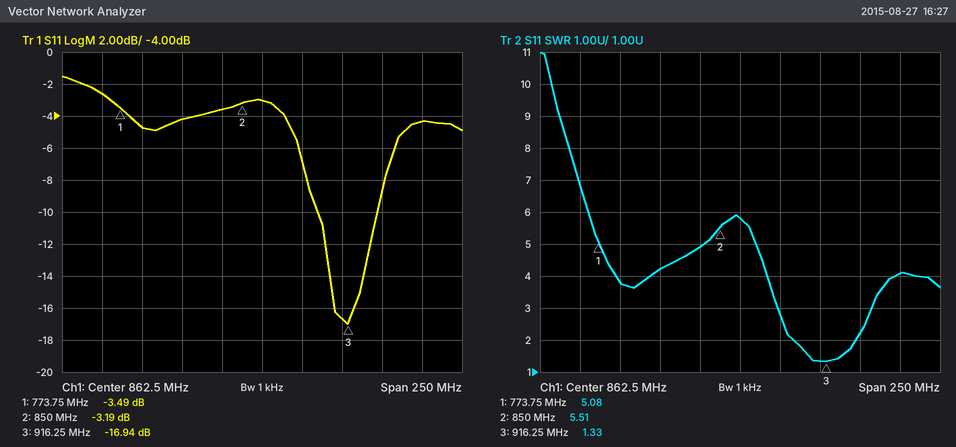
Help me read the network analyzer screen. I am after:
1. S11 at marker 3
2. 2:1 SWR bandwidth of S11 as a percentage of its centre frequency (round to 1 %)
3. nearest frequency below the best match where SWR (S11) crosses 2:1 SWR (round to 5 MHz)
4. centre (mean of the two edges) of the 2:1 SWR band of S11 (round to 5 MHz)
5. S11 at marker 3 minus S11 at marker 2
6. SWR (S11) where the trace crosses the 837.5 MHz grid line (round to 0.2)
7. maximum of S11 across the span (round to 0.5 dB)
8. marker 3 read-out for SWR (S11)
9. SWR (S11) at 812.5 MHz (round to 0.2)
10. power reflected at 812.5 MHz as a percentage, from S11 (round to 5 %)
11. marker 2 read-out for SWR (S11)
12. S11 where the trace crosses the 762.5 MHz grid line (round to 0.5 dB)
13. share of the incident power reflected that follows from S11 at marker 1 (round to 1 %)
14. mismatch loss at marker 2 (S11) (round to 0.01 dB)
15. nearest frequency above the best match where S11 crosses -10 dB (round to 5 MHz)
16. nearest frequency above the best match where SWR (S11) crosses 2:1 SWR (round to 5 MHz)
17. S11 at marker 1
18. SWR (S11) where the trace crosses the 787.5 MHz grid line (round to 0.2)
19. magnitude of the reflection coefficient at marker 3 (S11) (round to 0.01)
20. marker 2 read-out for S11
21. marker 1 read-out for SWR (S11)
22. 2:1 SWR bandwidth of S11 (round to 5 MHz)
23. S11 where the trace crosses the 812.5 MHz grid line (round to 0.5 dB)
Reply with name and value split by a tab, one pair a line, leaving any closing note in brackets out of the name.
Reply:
S11 at marker 3	-16.94 dB
2:1 SWR bandwidth of S11 as a percentage of its centre frequency	4 %
nearest frequency below the best match where SWR (S11) crosses 2:1 SWR	895 MHz
centre (mean of the two edges) of the 2:1 SWR band of S11	915 MHz
S11 at marker 3 minus S11 at marker 2	-13.75 dB
SWR (S11) where the trace crosses the 837.5 MHz grid line	5.0
maximum of S11 across the span	-1.5 dB
marker 3 read-out for SWR	1.33
SWR (S11) at 812.5 MHz	4.2
power reflected at 812.5 MHz as a percentage, from S11	40 %
marker 2 read-out for SWR	5.51
S11 where the trace crosses the 762.5 MHz grid line	-2.5 dB
share of the incident power reflected that follows from S11 at marker 1	45 %
mismatch loss at marker 2 (S11)	2.84 dB
nearest frequency above the best match where S11 crosses -10 dB	935 MHz
nearest frequency above the best match where SWR (S11) crosses 2:1 SWR	935 MHz
S11 at marker 1	-3.49 dB
SWR (S11) where the trace crosses the 787.5 MHz grid line	3.8
magnitude of the reflection coefficient at marker 3 (S11)	0.14
marker 2 read-out for S11	-3.19 dB
marker 1 read-out for SWR	5.08
2:1 SWR bandwidth of S11	40 MHz
S11 where the trace crosses the 812.5 MHz grid line	-4.0 dB
